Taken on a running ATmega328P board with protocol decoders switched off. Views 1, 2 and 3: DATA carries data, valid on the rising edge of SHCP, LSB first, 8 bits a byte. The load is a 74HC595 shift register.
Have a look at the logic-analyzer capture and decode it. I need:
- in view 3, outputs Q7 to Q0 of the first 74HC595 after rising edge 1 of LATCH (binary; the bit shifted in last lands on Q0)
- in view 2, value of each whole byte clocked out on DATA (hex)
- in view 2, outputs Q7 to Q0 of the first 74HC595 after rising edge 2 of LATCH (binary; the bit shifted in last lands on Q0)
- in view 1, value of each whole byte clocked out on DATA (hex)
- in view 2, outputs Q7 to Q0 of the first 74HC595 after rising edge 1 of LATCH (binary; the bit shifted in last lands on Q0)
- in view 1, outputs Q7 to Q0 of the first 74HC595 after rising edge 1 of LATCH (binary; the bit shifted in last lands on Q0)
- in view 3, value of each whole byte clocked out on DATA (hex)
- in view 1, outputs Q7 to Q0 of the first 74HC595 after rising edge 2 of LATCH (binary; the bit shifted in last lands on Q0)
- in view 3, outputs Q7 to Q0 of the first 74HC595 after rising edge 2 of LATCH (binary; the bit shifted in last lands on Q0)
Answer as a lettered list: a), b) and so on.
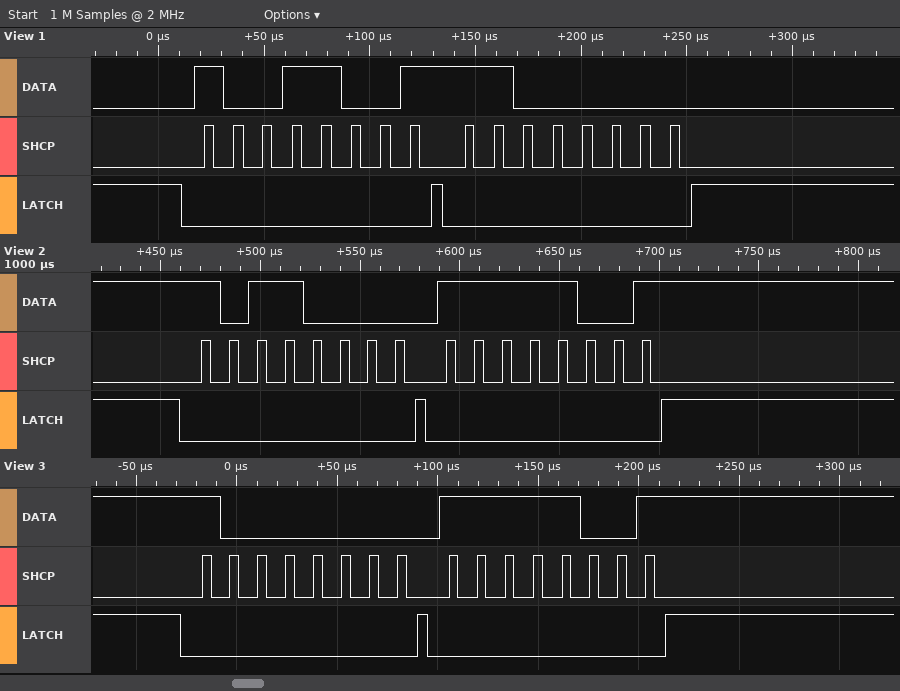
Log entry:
a) 10000000
b) 0D 9F
c) 11111001
d) 99 03
e) 10110000
f) 10011001
g) 01 9F
h) 11000000
i) 11111001
